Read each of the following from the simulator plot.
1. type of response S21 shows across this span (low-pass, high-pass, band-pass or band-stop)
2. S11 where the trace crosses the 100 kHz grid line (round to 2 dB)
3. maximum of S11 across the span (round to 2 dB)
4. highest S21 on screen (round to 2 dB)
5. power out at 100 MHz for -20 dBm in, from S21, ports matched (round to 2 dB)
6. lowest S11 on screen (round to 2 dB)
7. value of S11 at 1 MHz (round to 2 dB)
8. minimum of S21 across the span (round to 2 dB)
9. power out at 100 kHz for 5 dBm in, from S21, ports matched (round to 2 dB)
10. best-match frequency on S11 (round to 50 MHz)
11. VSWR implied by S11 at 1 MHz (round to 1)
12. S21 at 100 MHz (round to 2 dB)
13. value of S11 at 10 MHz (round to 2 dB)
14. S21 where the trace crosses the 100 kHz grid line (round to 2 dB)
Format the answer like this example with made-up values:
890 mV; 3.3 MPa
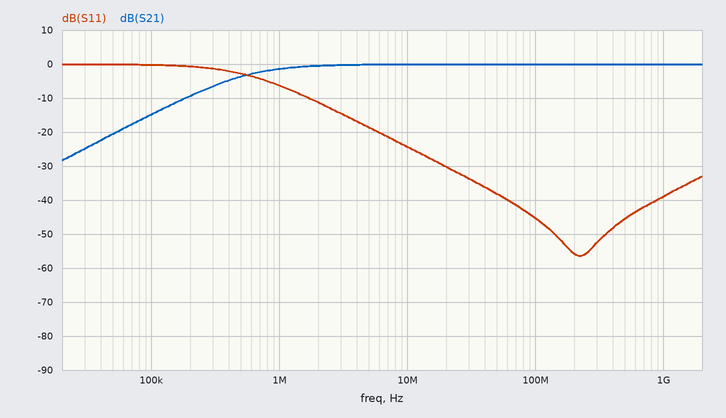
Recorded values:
high-pass; 0 dB; 0 dB; 0 dB; -20 dBm; -56 dB; -6 dB; -28 dB; -10 dBm; 200 MHz; 3; 0 dB; -24 dB; -14 dB
